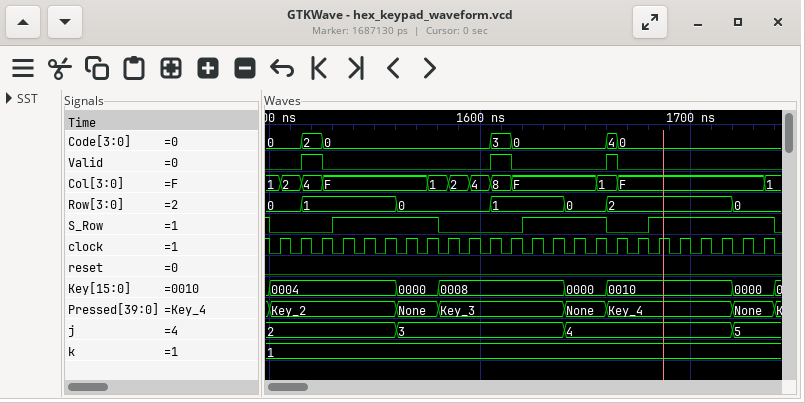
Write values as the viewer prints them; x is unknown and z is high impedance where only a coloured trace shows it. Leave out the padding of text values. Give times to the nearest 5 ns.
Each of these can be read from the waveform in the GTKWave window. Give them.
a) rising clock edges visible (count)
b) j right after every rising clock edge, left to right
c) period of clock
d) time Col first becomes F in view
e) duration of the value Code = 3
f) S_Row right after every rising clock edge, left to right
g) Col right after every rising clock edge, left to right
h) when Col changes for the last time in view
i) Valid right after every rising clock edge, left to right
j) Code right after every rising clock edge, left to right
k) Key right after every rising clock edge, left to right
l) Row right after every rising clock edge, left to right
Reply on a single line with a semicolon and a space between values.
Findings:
24; 2, 2, 2, 2, 2, 2, 3, 3, 3, 3, 3, 3, 3, 3, 4, 4, 4, 4, 4, 4, 4, 4, 5, 5; 10 ns; 1525 ns; 10 ns; 0 0 0 1 1 1 1 1 0 0 0 0 1 1 1 1 0 0 1 1 1 1 1 1; 2, 4, F, F, F, F, F, 1, 2, 4, 8, F, F, F, F, 1, F, F, F, F, F, F, F, 1; 1735 ns; 0 1 0 0 0 0 0 0 0 0 1 0 0 0 0 0 0 0 0 0 0 0 0 0; 0, 2, 0, 0, 0, 0, 0, 0, 0, 0, 3, 0, 0, 0, 0, 0, 0, 0, 0, 0, 0, 0, 0, 0; 0004, 0004, 0004, 0004, 0004, 0004, 0000, 0000, 0008, 0008, 0008, 0008, 0008, 0008, 0000, 0000, 0010, 0010, 0010, 0010, 0010, 0010, 0000, 0000; 0, 1, 1, 1, 1, 1, 0, 0, 0, 0, 1, 1, 1, 1, 0, 0, 2, 2, 2, 2, 2, 2, 0, 0
